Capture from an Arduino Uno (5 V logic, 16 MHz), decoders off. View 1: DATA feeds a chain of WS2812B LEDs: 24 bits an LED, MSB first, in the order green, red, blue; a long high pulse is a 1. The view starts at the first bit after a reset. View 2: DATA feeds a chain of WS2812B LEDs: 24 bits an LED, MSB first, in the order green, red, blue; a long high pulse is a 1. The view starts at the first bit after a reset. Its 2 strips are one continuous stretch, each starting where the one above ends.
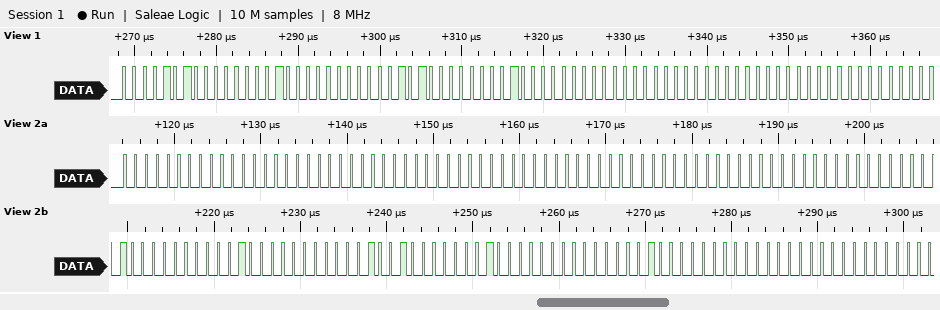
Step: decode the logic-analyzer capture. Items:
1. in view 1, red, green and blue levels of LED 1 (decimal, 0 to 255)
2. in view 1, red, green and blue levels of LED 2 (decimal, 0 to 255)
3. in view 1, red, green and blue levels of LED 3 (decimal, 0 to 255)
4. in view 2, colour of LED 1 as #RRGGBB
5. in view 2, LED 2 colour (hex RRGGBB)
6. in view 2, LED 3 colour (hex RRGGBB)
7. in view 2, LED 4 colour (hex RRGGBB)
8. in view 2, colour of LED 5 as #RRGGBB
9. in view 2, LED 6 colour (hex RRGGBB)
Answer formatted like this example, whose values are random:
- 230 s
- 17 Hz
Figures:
- 1, 10, 0
- 2, 20, 0
- 0, 0, 0
- #000000
- #000000
- #000000
- #010800
- #021200
- #000400
